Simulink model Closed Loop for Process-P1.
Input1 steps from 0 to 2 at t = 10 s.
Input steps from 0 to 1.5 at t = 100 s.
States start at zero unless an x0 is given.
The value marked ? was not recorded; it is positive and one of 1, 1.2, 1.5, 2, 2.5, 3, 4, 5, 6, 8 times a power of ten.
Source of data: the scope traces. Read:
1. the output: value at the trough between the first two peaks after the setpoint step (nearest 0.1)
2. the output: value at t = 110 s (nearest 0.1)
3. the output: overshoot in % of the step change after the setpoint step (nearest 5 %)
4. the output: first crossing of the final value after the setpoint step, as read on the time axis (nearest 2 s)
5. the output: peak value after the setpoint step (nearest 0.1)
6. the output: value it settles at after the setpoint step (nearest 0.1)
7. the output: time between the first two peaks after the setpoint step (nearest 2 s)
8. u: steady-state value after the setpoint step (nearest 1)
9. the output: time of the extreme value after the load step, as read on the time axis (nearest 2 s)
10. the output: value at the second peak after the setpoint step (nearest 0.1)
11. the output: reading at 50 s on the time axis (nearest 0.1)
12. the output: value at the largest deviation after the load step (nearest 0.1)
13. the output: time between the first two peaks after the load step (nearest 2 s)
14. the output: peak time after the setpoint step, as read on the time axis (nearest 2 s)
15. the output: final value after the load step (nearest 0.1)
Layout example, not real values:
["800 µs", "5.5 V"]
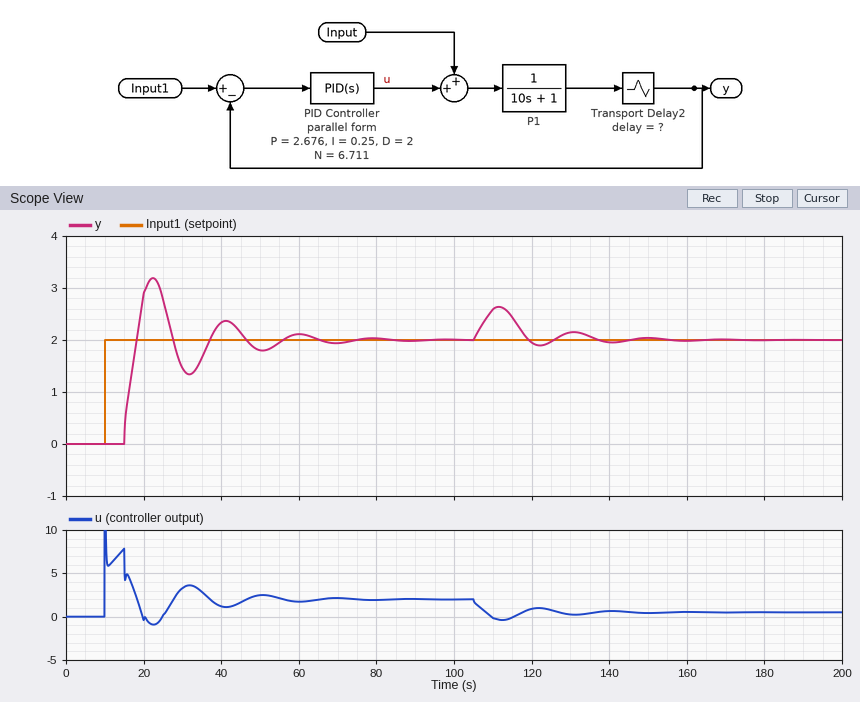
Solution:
["1.3", "2.6", "60 %", "18 s", "3.2", "2.0", "18 s", "2", "112 s", "2.4", "1.8", "2.6", "20 s", "22 s", "2.0"]
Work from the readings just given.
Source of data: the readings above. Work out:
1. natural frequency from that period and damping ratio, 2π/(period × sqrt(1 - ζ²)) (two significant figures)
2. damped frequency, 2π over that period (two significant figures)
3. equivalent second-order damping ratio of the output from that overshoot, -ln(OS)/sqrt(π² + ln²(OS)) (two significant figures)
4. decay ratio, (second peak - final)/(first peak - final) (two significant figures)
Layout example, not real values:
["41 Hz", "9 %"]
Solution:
["0.35 rad/s", "0.35 rad/s", "0.16", "0.33"]
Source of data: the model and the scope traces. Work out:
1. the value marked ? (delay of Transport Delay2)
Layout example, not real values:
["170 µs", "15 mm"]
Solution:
["5"]
